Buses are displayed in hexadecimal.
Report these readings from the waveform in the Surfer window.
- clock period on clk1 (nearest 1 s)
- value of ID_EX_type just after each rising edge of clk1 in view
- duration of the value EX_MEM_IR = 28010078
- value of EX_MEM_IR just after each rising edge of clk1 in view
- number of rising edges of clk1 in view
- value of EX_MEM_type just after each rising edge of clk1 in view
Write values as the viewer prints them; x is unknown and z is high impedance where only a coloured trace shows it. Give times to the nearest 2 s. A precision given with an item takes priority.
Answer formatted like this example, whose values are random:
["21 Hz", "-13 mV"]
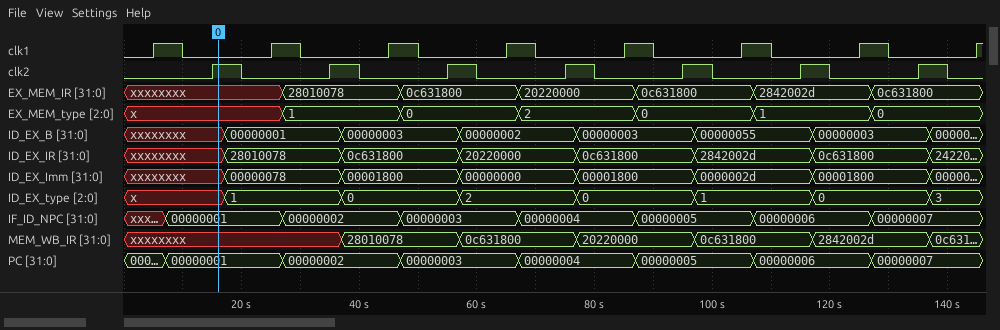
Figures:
["20 s", "x, 1, 0, 2, 0, 1, 0, 3", "20 s", "xxxxxxxx, xxxxxxxx, 28010078, 0c631800, 20220000, 0c631800, 2842002d, 0c631800", "8", "x, x, 1, 0, 2, 0, 1, 0"]
